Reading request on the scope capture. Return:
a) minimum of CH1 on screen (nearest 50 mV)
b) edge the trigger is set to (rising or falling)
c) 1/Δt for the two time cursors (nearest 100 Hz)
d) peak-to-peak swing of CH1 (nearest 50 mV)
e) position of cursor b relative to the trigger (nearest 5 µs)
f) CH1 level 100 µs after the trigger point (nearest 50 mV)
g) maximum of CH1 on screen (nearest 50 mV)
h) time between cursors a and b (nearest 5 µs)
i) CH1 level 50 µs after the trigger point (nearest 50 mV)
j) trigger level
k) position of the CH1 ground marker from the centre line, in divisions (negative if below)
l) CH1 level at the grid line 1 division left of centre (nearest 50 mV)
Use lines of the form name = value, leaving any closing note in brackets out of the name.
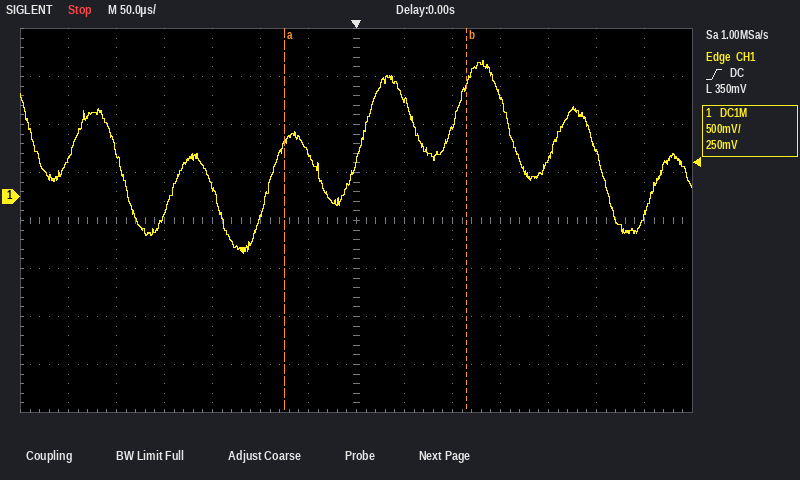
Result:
minimum of CH1 on screen = -600 mV
edge the trigger is set to = rising
1/Δt for the two time cursors = 5.3 kHz
peak-to-peak swing of CH1 = 2.00 V
position of cursor b relative to the trigger = +115 µs
CH1 level 100 µs after the trigger point = 700 mV
maximum of CH1 on screen = 1.40 V
time between cursors a and b = 190 µs
CH1 level 50 µs after the trigger point = 1.00 V
trigger level = 350 mV
position of the CH1 ground marker from the centre line, in divisions = +0.5 div
CH1 level at the grid line 1 division left of centre = 450 mV
